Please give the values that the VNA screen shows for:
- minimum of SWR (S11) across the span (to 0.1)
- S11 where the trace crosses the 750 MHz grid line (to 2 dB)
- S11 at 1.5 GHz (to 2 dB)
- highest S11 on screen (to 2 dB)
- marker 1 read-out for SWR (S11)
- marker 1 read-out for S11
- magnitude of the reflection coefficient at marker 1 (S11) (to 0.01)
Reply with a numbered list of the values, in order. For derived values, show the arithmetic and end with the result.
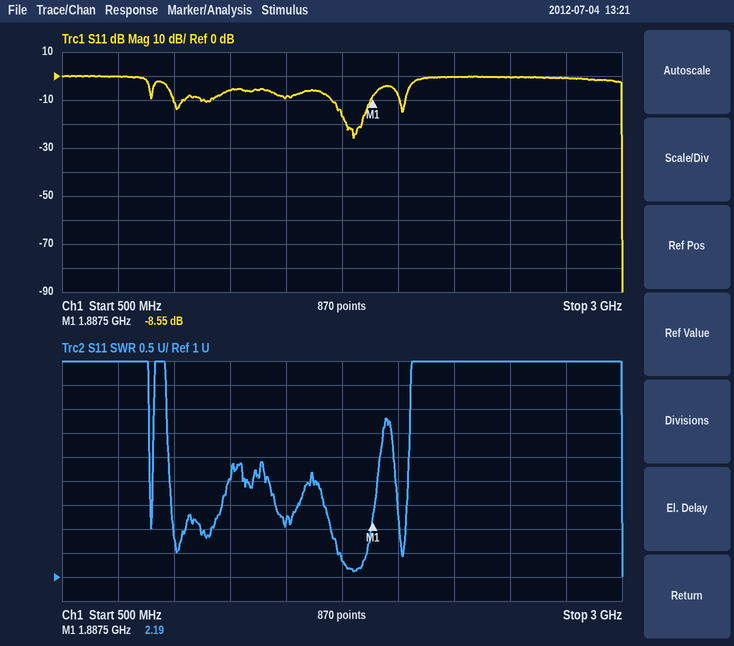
1. 1.0
2. 0 dB
3. -8 dB
4. 0 dB
5. 2.19
6. -8.55 dB
7. 10^(-8.55/20) ≈ 0.37
